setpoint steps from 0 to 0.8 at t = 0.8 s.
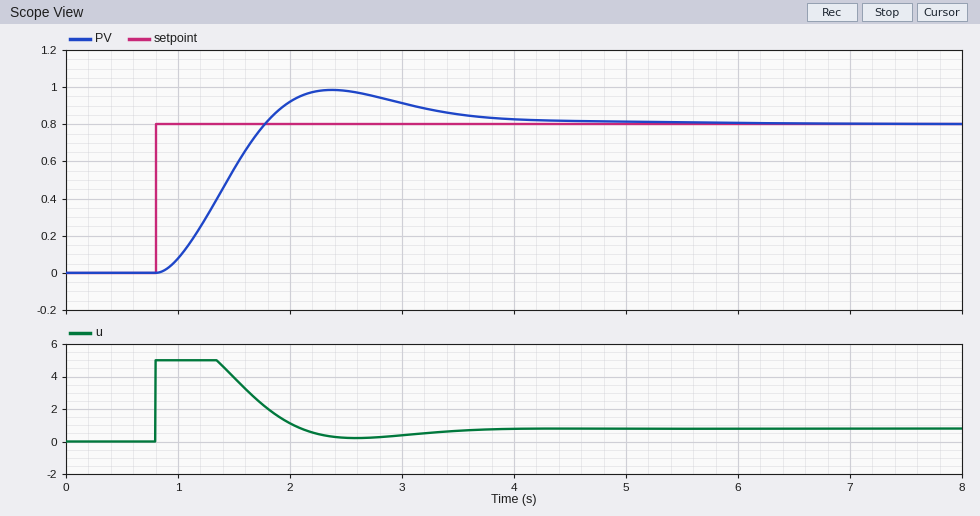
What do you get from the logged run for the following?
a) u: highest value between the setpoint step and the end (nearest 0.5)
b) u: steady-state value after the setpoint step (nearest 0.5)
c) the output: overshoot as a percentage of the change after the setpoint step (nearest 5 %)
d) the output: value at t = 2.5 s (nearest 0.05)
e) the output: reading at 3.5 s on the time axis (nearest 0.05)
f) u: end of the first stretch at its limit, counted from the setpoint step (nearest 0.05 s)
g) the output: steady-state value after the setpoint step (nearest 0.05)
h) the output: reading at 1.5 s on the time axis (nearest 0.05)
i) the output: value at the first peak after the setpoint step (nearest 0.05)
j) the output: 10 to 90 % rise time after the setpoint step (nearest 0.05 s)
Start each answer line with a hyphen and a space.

- 5.0
- 1.0
- 25 %
- 1.00
- 0.85
- 0.55 s
- 0.80
- 0.55
- 1.00
- 0.65 s
